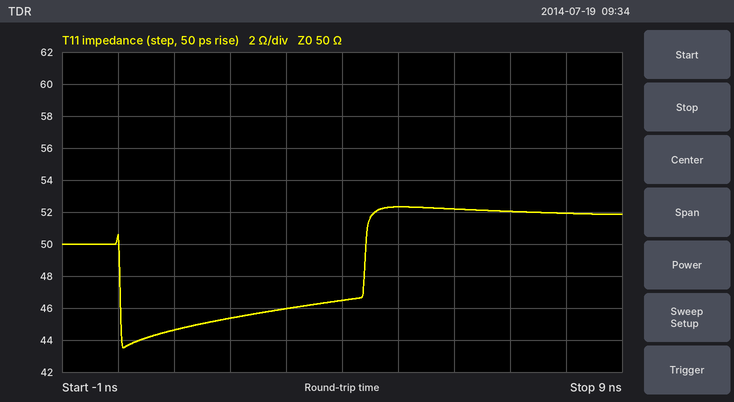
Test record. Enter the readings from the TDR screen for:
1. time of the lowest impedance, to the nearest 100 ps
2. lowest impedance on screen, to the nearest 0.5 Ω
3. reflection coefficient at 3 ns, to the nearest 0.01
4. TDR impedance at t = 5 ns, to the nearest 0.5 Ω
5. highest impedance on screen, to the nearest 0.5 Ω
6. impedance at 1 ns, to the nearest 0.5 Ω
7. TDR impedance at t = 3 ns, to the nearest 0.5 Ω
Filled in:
100 ps
43.5 Ω
-0.04
52.5 Ω
52.5 Ω
44.5 Ω
46.0 Ω
